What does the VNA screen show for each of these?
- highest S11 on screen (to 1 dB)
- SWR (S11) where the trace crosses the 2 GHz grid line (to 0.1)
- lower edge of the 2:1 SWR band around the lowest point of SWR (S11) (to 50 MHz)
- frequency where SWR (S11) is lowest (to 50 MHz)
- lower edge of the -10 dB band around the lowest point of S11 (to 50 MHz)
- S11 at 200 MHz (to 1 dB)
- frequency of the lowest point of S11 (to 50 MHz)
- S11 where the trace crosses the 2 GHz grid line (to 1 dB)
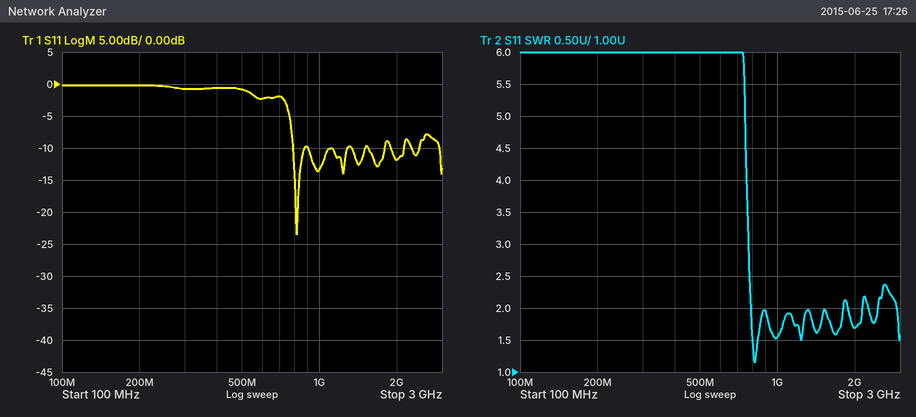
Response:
0 dB
1.7
800 MHz
800 MHz
800 MHz
0 dB
800 MHz
-12 dB
